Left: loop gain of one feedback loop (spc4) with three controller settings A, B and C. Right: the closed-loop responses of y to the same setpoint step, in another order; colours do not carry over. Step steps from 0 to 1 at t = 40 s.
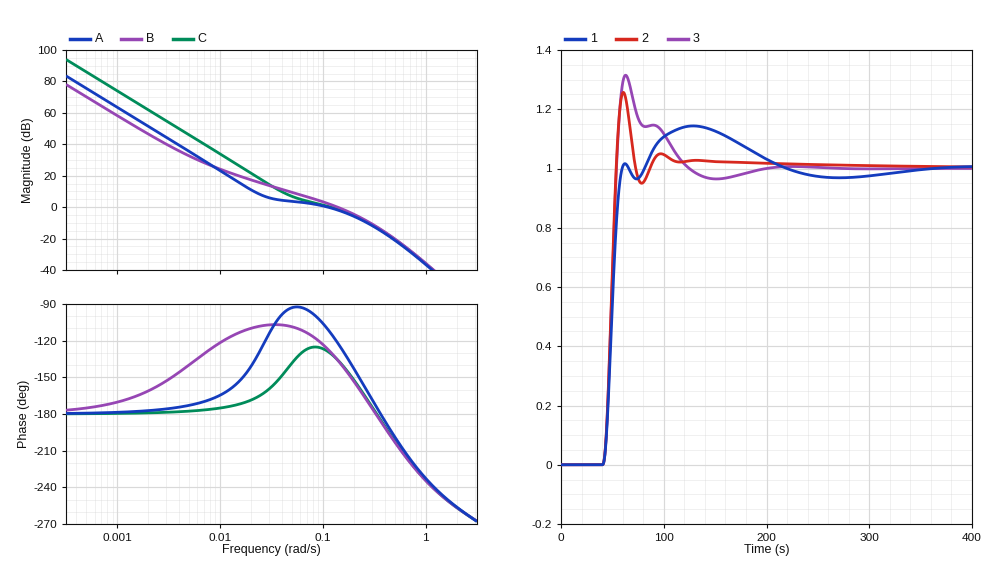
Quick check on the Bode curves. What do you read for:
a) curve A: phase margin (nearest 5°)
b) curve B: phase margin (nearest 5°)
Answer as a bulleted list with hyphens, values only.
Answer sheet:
- 70°
- 45°
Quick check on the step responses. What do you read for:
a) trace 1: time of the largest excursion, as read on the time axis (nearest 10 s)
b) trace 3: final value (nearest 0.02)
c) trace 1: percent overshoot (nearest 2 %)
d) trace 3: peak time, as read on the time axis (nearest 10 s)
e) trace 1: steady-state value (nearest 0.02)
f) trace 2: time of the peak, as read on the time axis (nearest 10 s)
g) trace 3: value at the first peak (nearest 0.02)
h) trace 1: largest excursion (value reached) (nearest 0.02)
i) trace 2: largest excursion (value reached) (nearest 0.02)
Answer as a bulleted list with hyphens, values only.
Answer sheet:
- 130 s
- 1.00
- 14 %
- 60 s
- 1.00
- 60 s
- 1.32
- 1.14
- 1.26
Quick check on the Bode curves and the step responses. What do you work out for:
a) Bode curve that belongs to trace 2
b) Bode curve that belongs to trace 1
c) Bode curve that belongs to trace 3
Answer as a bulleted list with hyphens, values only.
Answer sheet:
- B
- A
- C
